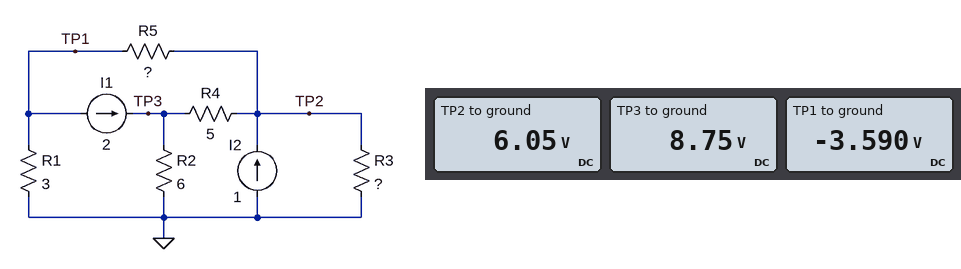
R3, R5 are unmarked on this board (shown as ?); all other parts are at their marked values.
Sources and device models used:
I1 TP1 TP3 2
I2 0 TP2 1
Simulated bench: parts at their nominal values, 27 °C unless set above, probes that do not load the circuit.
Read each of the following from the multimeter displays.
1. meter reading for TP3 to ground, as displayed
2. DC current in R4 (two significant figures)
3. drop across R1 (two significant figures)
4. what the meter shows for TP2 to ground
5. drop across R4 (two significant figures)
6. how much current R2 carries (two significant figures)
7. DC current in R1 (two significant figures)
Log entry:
8.75 V
540 mA
3.6 V
6.05 V
2.7 V
1.5 A
1.2 A
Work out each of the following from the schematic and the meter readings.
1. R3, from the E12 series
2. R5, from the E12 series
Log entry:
8.2 Ω
12 Ω
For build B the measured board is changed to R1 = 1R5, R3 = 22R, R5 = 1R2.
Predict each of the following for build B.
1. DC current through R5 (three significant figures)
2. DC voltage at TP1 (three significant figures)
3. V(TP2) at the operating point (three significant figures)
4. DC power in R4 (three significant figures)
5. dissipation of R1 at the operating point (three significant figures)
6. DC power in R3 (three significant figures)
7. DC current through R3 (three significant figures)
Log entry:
1.83 A
-259 mV
1.93 V
4.19 W
44.8 mW
170 mW
87.9 mA
